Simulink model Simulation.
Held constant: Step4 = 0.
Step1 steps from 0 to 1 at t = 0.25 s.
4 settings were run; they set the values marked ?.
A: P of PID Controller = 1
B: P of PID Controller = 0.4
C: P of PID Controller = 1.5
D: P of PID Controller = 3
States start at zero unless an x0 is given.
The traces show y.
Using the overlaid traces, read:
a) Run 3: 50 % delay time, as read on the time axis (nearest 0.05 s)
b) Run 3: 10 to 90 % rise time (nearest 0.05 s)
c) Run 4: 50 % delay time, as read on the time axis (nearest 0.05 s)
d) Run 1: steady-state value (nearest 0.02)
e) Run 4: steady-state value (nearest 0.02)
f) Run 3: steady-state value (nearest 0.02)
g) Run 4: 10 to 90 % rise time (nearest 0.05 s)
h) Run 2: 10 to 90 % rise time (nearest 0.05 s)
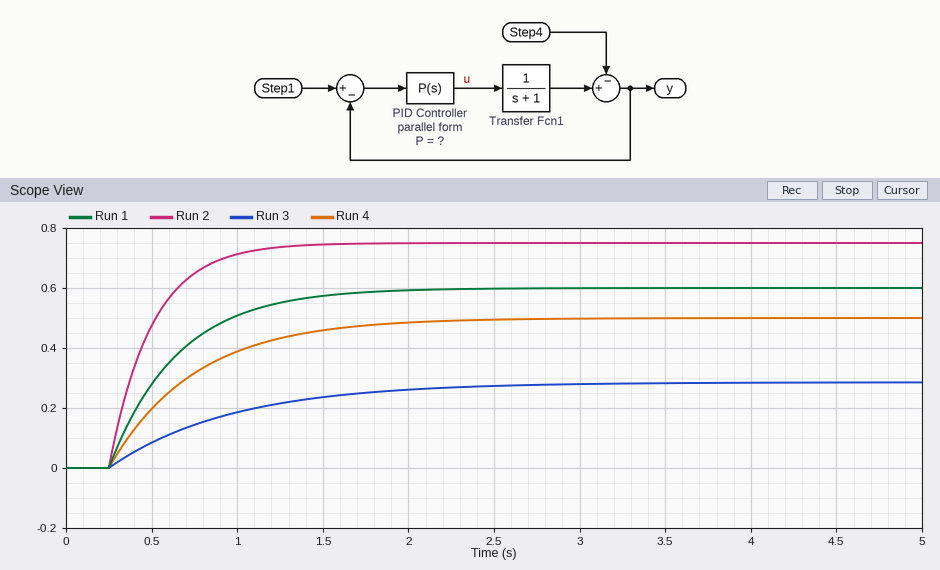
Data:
0.75 s
1.55 s
0.60 s
0.60
0.50
0.28
1.10 s
0.55 s
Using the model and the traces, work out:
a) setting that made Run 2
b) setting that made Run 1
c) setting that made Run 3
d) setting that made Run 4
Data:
D
C
B
A
